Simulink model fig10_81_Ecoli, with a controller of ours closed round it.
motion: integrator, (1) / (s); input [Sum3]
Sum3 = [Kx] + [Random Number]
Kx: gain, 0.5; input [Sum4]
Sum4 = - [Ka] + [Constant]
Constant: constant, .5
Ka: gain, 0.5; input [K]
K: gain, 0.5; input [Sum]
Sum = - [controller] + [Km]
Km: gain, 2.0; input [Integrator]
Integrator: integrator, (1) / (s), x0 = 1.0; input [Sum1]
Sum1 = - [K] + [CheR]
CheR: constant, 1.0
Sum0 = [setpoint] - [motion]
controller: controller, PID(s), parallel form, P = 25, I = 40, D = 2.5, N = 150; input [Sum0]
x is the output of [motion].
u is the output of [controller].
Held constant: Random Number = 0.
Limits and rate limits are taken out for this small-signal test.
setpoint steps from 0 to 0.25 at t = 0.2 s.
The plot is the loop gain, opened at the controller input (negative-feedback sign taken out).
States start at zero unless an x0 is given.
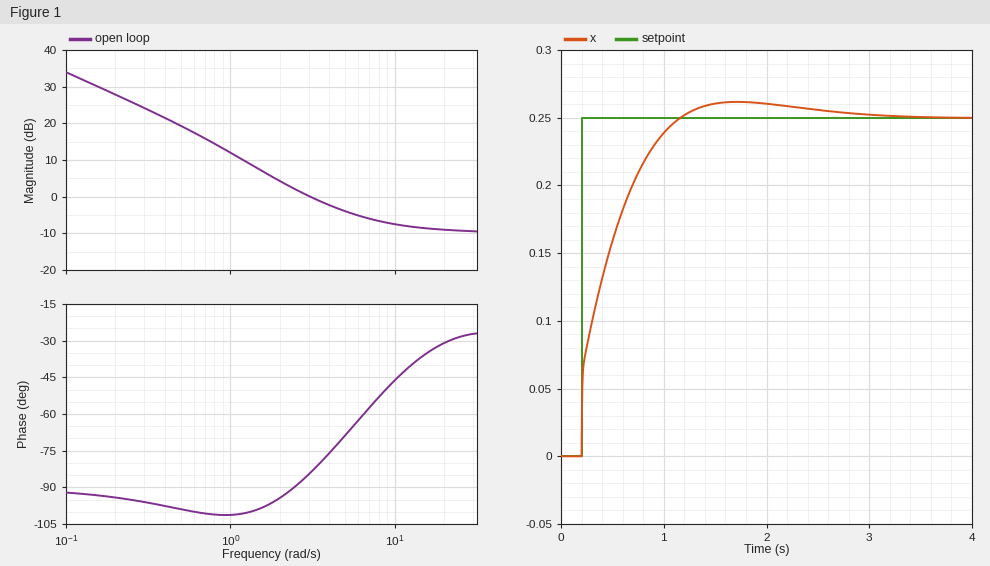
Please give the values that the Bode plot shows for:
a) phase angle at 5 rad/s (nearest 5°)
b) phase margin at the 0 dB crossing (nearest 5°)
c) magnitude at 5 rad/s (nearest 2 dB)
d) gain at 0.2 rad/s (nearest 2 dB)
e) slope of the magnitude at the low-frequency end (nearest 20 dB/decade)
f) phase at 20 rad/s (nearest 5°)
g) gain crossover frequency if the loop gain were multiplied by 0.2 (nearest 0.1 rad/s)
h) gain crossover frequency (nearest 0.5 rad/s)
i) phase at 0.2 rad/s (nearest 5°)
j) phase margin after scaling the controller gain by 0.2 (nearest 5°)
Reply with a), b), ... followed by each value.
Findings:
a) -70°
b) 95°
c) -4 dB
d) 28 dB
e) -20 dB/decade
f) -30°
g) 0.8 rad/s
h) 3.0 rad/s
i) -95°
j) 80°
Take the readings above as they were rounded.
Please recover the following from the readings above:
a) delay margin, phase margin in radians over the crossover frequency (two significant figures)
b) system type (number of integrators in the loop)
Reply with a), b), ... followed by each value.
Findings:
a) 0.55 s
b) 1
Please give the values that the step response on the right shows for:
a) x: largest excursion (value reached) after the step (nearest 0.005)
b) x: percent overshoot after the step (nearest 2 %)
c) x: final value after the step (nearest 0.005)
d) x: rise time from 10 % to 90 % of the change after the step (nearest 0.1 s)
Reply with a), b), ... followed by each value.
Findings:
a) 0.260
b) 4 %
c) 0.250
d) 0.7 s
